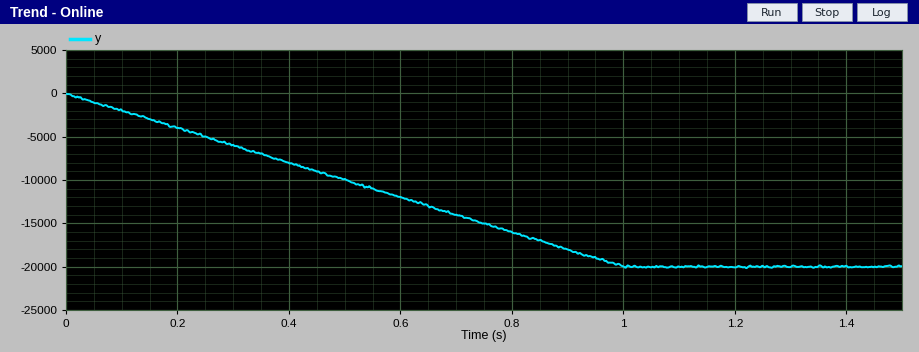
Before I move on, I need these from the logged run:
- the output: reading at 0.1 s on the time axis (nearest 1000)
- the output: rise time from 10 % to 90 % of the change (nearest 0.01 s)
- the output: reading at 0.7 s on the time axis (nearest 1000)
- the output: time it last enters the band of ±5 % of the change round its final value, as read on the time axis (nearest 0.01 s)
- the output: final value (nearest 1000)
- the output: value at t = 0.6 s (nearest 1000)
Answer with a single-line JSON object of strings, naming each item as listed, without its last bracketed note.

{"the output: reading at 0.1 s on the time axis": "-2000", "the output: rise time from 10 % to 90 % of the change": "0.80 s", "the output: reading at 0.7 s on the time axis": "-14000", "the output: time it last enters the band of ±5 % of the change round its final value, as read on the time axis": "0.95 s", "the output: final value": "-20000", "the output: value at t = 0.6 s": "-12000"}
